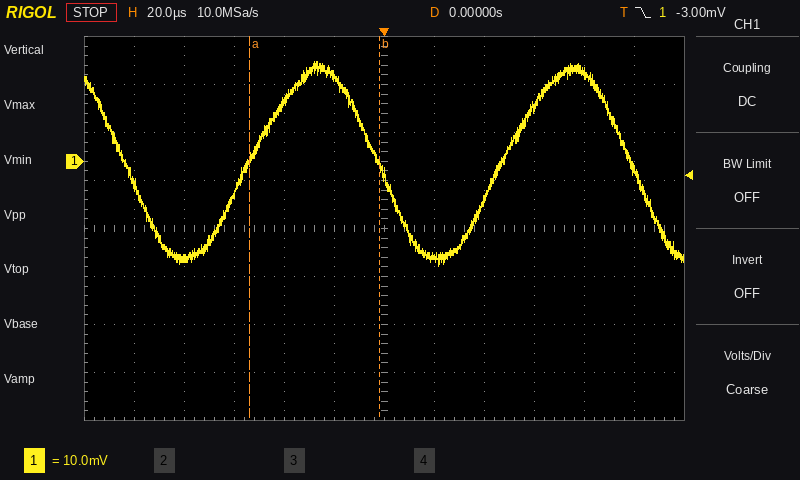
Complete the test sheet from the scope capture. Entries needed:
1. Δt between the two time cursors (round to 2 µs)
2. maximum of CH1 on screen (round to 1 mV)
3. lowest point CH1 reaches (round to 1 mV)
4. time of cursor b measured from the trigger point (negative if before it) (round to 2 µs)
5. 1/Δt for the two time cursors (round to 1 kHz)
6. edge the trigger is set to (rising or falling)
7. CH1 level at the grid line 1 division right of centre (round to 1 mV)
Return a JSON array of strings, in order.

["52 µs", "21 mV", "-22 mV", "-2 µs", "19 kHz", "falling", "-20 mV"]
